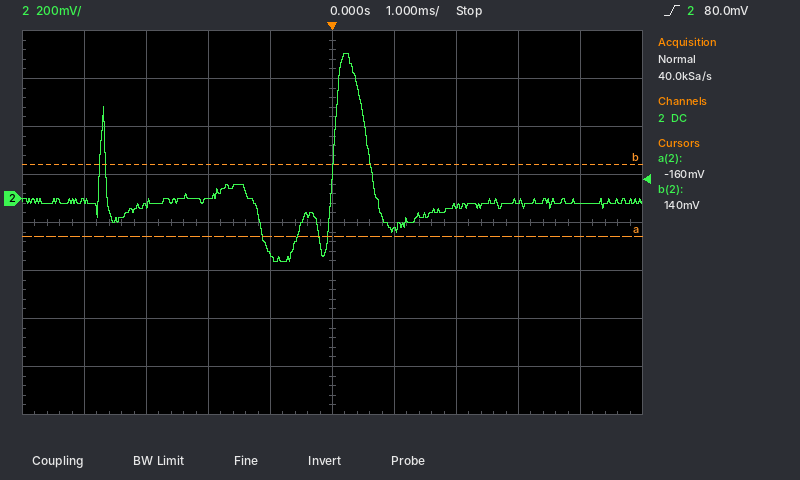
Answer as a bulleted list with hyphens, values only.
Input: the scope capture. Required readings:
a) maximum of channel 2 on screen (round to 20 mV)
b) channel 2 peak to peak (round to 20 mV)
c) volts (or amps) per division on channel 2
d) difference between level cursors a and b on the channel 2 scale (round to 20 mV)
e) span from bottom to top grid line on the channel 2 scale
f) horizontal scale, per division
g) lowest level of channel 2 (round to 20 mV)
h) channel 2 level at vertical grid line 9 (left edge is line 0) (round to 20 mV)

- 600 mV
- 860 mV
- 200 mV
- 300 mV
- 1.6 V
- 1 ms
- -260 mV
- -20 mV
